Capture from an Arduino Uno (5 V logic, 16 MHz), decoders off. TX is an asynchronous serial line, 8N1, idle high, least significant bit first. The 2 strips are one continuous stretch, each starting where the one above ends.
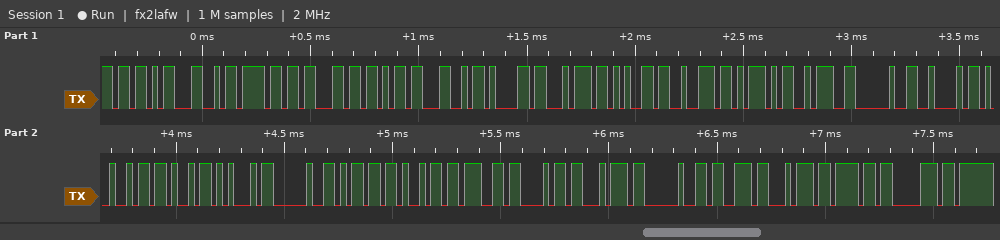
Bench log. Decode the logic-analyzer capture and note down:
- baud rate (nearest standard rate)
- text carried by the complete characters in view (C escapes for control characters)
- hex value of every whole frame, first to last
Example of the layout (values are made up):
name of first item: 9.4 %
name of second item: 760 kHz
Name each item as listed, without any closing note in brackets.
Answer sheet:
baud rate: 38400 baud
text carried by the complete characters in view: "[LockLater]: BIKE might stop"
hex value of every whole frame, first to last: 5B 4C 6F 63 6B 4C 61 74 65 72 5D 3A 20 42 49 4B 45 20 6D 69 67 68 74 20 73 74 6F 70
